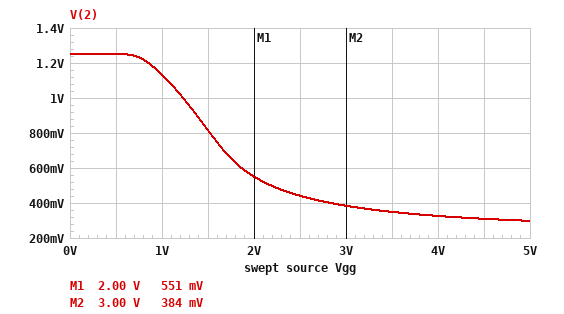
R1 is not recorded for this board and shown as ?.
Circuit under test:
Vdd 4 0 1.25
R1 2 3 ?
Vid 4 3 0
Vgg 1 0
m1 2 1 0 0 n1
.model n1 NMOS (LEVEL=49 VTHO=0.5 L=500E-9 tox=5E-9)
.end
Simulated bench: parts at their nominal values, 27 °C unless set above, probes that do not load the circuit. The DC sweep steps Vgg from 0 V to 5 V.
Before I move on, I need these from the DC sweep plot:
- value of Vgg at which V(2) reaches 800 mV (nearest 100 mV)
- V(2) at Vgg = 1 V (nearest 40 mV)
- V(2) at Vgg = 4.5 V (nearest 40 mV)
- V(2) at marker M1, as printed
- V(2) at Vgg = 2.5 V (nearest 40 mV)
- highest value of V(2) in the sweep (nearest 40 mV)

1.5 V
1.12 V
320 mV
551 mV
440 mV
1.24 V
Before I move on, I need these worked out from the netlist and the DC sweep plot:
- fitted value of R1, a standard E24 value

750 Ω
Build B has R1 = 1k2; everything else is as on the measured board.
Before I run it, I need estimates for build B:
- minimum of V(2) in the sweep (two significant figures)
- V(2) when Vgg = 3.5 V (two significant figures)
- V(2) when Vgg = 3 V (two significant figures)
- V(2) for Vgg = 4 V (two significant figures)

200 mV
230 mV
260 mV
220 mV
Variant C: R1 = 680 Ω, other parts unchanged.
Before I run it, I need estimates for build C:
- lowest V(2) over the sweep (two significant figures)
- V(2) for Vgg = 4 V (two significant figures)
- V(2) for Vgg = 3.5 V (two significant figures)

320 mV
350 mV
380 mV
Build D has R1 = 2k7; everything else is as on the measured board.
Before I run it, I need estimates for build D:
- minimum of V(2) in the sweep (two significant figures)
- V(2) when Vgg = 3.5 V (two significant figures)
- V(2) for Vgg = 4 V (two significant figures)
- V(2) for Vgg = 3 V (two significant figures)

94 mV
110 mV
100 mV
120 mV
